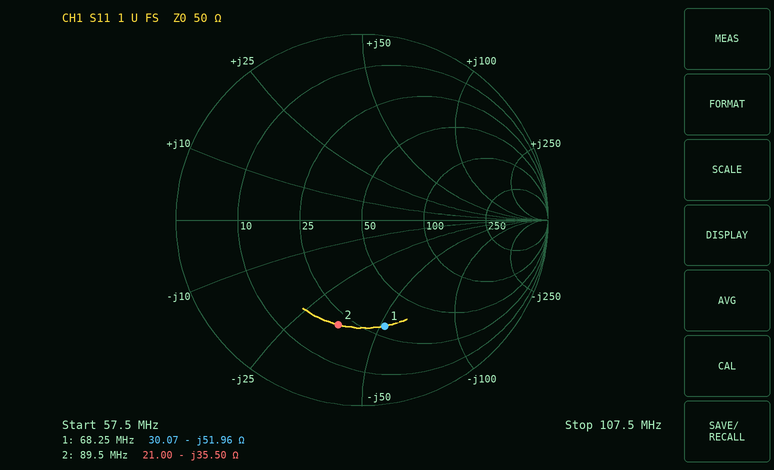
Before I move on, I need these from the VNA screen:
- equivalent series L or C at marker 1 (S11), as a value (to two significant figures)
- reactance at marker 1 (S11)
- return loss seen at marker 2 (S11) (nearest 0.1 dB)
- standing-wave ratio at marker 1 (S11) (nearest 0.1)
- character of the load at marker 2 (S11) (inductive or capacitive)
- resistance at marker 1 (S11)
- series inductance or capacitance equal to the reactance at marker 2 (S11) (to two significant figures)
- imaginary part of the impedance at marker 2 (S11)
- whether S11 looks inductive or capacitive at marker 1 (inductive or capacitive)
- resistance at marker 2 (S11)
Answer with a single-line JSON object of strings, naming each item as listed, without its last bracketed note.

{"equivalent series L or C at marker 1 (S11), as a value": "45 pF", "reactance at marker 1": "-51.96 Ω", "return loss seen at marker 2 (S11)": "4.8 dB", "standing-wave ratio at marker 1 (S11)": "3.8", "character of the load at marker 2 (S11)": "capacitive", "resistance at marker 1": "30.07 Ω", "series inductance or capacitance equal to the reactance at marker 2 (S11)": "50 pF", "imaginary part of the impedance at marker 2": "-35.50 Ω", "whether S11 looks inductive or capacitive at marker 1": "capacitive", "resistance at marker 2": "21.00 Ω"}
